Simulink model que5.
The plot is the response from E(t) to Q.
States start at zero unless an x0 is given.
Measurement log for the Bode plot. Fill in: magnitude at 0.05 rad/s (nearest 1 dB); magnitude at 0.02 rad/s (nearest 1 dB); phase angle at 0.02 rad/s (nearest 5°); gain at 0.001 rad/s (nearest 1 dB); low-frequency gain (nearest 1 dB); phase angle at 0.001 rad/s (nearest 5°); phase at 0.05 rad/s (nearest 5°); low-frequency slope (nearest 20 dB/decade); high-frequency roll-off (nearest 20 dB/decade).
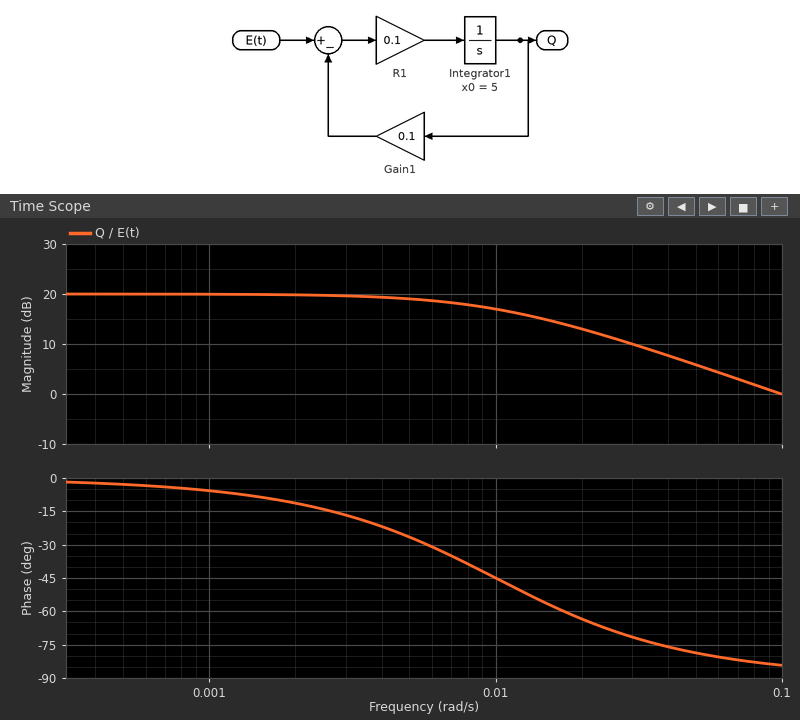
6 dB
13 dB
-65°
20 dB
20 dB
-5°
-80°
0 dB/decade
-20 dB/decade
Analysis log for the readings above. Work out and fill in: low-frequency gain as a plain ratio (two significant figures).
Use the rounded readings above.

10
